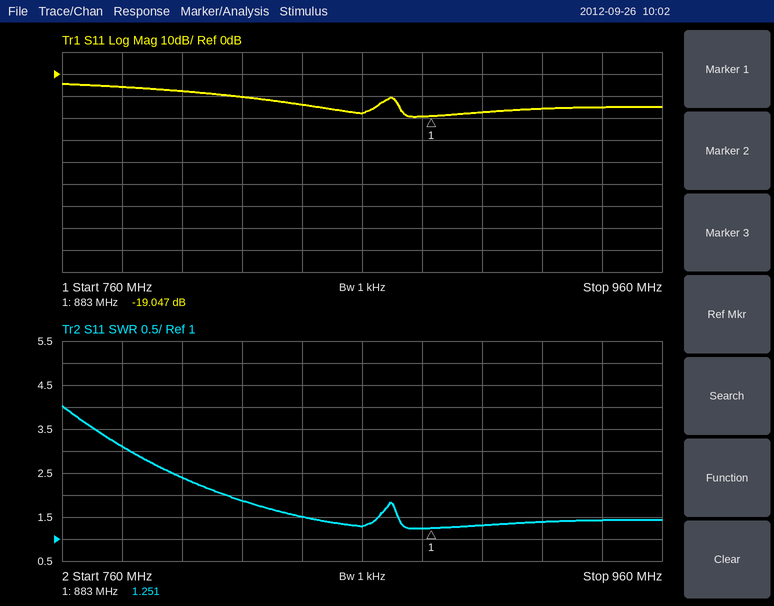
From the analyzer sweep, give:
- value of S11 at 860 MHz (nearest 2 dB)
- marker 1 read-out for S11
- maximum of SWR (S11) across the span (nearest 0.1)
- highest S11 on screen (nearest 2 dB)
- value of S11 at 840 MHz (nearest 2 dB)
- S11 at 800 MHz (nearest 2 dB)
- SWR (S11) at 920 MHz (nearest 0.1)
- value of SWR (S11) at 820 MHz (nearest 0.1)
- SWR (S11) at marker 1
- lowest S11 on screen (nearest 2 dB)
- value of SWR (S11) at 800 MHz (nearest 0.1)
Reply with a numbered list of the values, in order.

1. -18 dB
2. -19.047 dB
3. 4.0
4. -4 dB
5. -14 dB
6. -8 dB
7. 1.4
8. 1.9
9. 1.251
10. -20 dB
11. 2.4
